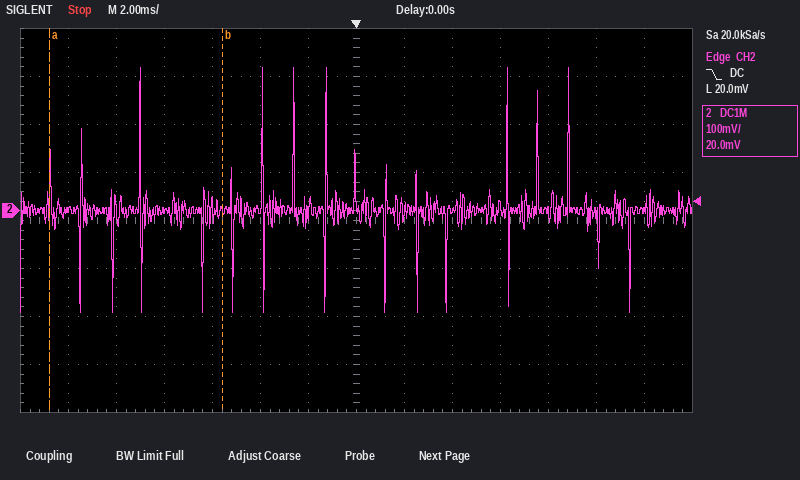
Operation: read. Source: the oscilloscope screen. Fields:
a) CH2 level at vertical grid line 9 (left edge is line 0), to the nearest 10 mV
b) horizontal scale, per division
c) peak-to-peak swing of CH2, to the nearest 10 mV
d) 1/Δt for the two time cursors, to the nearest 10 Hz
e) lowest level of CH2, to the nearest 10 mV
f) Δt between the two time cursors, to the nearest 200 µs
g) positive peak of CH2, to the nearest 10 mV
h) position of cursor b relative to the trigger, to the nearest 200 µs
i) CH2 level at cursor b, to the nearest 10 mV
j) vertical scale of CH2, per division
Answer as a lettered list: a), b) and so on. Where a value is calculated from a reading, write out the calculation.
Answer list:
a) 0 mV
b) 2 ms
c) 300 mV − (-210 mV) = 510 mV
d) 1 / 7.2 ms ≈ 140 Hz
e) -210 mV
f) 7.2 ms
g) 300 mV
h) -5.6 ms
i) 0 mV
j) 100 mV
